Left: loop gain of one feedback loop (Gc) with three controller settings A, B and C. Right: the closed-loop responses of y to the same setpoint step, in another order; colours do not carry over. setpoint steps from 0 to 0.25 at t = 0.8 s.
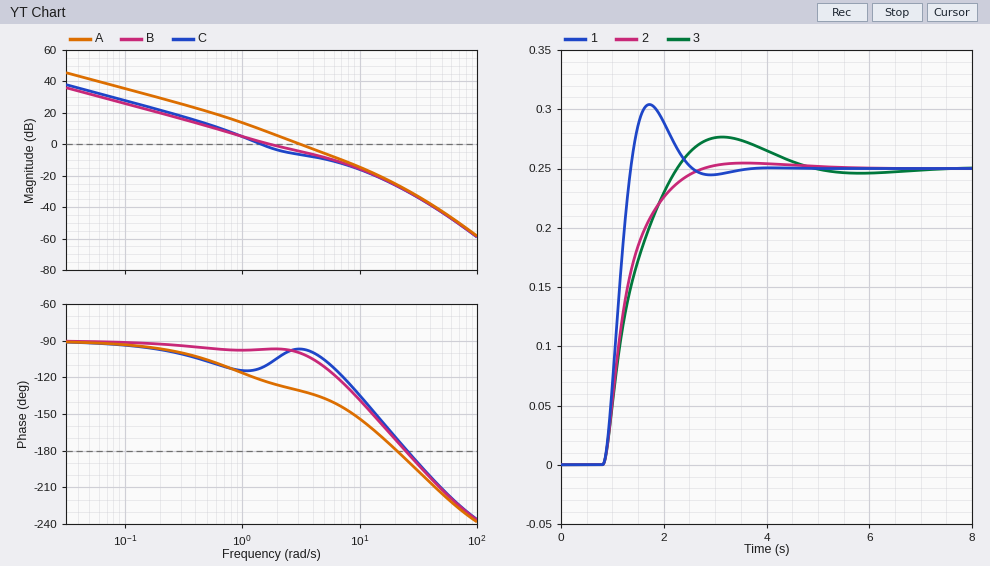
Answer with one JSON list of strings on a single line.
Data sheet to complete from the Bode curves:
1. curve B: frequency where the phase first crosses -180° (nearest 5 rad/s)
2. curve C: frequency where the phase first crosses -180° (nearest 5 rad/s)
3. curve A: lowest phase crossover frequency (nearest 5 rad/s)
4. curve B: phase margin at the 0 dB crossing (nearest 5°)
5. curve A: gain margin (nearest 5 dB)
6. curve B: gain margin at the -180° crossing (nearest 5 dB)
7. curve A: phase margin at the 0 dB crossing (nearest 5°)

["25 rad/s", "25 rad/s", "20 rad/s", "85°", "25 dB", "30 dB", "50°"]
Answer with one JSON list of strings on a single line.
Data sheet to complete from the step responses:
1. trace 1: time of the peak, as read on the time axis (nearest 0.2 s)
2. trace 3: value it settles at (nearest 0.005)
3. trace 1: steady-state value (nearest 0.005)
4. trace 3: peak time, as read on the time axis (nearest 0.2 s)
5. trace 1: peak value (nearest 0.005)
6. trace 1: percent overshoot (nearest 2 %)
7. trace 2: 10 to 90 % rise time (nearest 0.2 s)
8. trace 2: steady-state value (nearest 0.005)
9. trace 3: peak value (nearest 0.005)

["1.8 s", "0.250", "0.250", "3.2 s", "0.305", "22 %", "1.0 s", "0.250", "0.275"]
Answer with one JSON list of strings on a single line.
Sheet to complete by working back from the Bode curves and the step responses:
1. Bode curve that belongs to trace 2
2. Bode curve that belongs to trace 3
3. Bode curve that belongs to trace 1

["B", "C", "A"]
